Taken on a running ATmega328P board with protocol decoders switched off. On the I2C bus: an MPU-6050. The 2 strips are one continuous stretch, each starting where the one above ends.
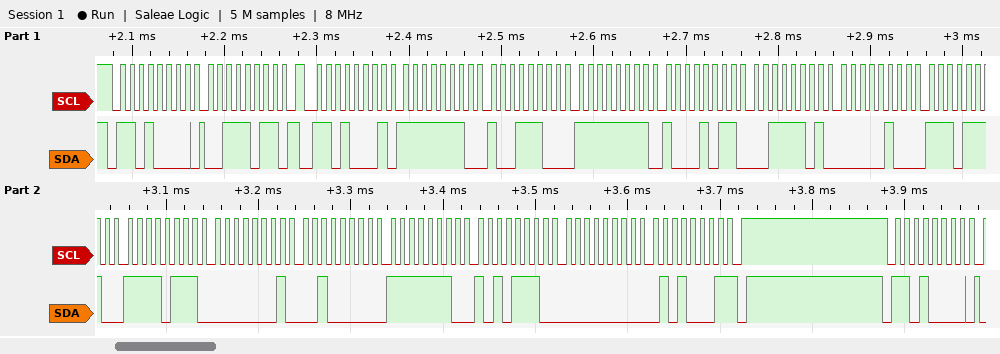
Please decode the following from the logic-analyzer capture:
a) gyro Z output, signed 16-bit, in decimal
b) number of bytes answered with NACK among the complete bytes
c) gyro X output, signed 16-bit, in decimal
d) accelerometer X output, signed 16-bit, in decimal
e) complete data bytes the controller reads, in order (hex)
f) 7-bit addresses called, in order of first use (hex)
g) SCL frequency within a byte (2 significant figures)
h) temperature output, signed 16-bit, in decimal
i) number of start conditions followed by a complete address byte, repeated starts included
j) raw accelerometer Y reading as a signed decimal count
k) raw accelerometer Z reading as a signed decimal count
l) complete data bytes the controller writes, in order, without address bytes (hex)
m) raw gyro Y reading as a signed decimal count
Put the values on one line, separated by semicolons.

81; 1; 288; -356; FE 9C FF 8B 3D 04 EE F7 01 20 FE AE 00 51; 0x68; 100 kHz; -4361; 3; -117; 15620; 3B; -338
